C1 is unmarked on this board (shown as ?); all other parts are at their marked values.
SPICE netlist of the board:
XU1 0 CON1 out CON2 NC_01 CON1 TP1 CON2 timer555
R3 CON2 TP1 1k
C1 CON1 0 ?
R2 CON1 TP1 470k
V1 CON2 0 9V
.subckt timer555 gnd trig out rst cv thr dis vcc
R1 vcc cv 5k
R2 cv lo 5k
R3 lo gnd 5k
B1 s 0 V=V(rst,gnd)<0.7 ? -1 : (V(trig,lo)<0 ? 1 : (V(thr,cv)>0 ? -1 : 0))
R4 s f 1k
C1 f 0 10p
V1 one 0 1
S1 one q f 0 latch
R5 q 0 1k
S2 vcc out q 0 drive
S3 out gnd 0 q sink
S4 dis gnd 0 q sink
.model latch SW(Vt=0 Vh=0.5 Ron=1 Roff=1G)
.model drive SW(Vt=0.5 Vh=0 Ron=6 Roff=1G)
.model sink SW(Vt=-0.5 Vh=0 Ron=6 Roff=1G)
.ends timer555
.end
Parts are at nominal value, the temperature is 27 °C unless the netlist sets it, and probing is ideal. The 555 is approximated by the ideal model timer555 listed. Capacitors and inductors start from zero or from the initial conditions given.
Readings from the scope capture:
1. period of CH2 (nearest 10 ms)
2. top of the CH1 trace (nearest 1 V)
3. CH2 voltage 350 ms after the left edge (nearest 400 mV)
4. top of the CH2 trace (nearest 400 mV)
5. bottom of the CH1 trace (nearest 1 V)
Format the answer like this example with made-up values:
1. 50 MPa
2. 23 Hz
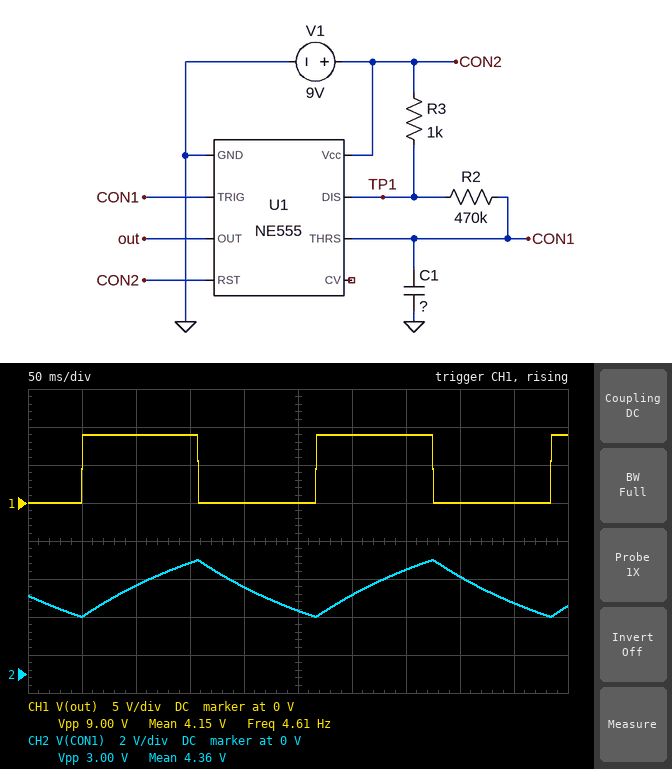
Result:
1. 220 ms
2. 9 V
3. 5.6 V
4. 6.0 V
5. 0 V
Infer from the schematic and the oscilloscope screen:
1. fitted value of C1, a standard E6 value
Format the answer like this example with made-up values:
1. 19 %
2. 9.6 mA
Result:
1. 330 nF
